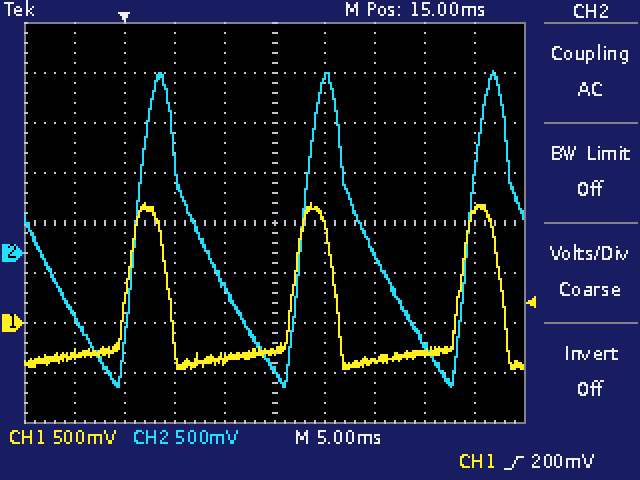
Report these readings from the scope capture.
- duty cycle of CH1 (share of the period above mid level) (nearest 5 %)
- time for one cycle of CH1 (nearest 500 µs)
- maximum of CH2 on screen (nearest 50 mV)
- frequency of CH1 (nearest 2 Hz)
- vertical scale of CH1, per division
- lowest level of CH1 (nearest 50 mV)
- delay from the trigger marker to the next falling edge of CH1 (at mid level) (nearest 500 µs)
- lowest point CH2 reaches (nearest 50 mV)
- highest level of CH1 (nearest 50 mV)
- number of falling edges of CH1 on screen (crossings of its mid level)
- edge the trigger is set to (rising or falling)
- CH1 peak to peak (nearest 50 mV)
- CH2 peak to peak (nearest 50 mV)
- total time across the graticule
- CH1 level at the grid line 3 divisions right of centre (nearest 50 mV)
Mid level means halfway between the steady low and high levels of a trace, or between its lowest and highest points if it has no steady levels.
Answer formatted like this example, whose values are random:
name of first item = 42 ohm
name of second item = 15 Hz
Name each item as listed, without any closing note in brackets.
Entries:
duty cycle of CH1 (share of the period above mid level) = 25 %
time for one cycle of CH1 = 16.5 ms
maximum of CH2 on screen = 1.80 V
frequency of CH1 = 60 Hz
vertical scale of CH1, per division = 500 mV
lowest level of CH1 = -450 mV
delay from the trigger marker to the next falling edge of CH1 (at mid level) = 4.5 ms
lowest point CH2 reaches = -1.35 V
highest level of CH1 = 1.20 V
number of falling edges of CH1 on screen = 3
edge the trigger is set to = rising
CH1 peak to peak = 1.65 V
CH2 peak to peak = 3.15 V
total time across the graticule = 50 ms
CH1 level at the grid line 3 divisions right of centre = -300 mV
